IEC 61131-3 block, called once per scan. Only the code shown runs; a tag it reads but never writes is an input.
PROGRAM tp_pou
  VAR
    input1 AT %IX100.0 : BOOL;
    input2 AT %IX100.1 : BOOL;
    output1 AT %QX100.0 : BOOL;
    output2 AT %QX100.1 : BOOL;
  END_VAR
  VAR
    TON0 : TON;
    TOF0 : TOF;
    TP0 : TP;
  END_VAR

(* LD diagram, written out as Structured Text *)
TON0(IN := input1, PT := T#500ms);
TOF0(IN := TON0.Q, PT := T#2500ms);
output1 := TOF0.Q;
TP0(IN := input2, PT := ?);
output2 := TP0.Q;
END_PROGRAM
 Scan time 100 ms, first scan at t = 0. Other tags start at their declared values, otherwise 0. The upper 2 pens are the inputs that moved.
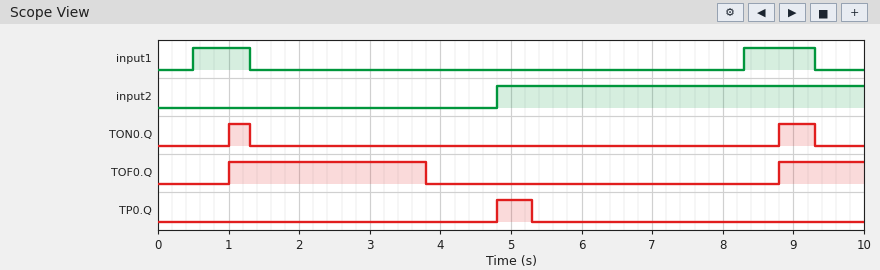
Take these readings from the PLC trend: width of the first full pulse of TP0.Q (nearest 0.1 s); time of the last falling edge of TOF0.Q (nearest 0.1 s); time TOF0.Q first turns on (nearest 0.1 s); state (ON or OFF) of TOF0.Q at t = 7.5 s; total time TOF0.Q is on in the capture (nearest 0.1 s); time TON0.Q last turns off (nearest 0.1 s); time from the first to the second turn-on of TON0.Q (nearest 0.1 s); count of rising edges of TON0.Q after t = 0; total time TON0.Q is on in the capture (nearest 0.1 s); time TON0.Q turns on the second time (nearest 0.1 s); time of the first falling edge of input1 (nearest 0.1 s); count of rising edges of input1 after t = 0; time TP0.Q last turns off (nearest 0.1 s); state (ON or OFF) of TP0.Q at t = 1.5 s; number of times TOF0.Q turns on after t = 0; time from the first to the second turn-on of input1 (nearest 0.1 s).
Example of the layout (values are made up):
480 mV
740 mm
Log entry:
0.5 s
3.8 s
1.0 s
OFF
4.0 s
9.3 s
7.8 s
2
0.8 s
8.8 s
1.3 s
2
5.3 s
OFF
2
7.8 s
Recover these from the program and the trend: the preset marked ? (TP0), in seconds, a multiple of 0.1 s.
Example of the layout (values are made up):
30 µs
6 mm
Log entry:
0.5 s
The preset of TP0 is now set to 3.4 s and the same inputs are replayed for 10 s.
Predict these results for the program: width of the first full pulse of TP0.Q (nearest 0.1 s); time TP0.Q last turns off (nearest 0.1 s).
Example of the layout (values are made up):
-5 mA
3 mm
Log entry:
3.4 s
8.2 s
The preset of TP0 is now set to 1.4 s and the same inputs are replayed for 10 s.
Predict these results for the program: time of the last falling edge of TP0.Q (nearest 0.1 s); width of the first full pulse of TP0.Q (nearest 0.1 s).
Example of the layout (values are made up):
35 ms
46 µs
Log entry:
6.2 s
1.4 s
